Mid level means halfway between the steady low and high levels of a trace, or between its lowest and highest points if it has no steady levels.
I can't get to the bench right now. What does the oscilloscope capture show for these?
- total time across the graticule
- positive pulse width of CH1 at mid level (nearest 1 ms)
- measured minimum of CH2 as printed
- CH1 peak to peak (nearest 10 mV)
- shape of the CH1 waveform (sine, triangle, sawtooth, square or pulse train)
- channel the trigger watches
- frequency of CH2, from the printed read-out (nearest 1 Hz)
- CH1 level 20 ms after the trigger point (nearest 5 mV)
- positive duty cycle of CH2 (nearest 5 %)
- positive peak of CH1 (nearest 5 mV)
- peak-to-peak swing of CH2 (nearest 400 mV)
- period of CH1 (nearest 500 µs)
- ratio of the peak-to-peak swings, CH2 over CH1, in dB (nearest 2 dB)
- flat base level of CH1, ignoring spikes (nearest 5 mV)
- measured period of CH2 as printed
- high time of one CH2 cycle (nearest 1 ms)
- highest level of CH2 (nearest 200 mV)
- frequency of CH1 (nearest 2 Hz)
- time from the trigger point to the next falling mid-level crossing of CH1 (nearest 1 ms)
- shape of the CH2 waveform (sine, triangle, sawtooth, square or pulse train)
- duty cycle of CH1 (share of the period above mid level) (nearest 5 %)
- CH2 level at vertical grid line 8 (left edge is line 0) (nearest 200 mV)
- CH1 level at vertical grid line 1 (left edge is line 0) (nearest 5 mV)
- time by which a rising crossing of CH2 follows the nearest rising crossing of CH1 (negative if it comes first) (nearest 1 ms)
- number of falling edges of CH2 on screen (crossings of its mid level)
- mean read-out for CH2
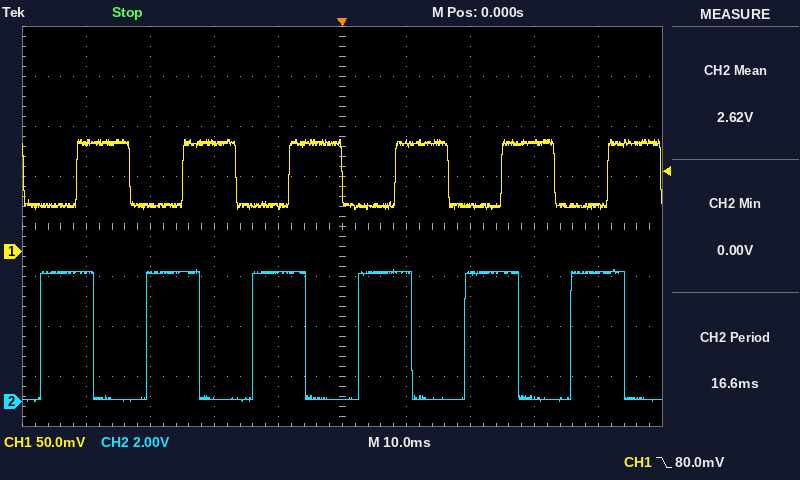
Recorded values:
100 ms
8 ms
0.00 V
70 mV
square
CH1
60 Hz
45 mV
50 %
110 mV
5.2 V
16.5 ms
38 dB
45 mV
16.6 ms
8 ms
5.2 V
60 Hz
17 ms
square
50 %
200 mV
110 mV
-6 ms
6
2.62 V
